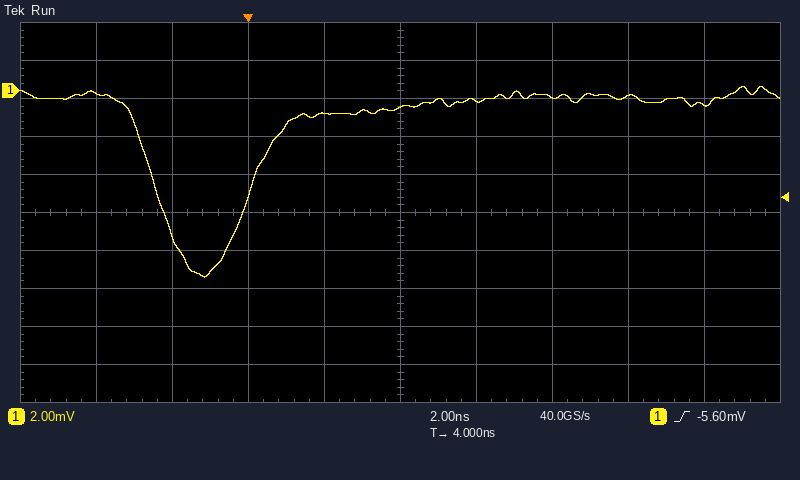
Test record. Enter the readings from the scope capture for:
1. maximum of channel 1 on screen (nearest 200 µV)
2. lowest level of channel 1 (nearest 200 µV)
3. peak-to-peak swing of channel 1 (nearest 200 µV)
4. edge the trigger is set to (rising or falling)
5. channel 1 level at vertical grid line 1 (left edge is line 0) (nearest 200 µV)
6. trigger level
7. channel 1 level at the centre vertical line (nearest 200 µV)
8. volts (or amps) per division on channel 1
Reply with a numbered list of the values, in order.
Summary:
1. 200 µV
2. -9.8 mV
3. 10.0 mV
4. rising
5. -200 µV
6. -5.60 mV
7. -800 µV
8. 2 mV
